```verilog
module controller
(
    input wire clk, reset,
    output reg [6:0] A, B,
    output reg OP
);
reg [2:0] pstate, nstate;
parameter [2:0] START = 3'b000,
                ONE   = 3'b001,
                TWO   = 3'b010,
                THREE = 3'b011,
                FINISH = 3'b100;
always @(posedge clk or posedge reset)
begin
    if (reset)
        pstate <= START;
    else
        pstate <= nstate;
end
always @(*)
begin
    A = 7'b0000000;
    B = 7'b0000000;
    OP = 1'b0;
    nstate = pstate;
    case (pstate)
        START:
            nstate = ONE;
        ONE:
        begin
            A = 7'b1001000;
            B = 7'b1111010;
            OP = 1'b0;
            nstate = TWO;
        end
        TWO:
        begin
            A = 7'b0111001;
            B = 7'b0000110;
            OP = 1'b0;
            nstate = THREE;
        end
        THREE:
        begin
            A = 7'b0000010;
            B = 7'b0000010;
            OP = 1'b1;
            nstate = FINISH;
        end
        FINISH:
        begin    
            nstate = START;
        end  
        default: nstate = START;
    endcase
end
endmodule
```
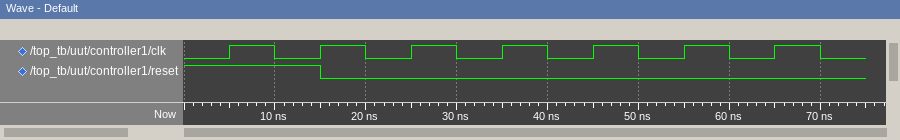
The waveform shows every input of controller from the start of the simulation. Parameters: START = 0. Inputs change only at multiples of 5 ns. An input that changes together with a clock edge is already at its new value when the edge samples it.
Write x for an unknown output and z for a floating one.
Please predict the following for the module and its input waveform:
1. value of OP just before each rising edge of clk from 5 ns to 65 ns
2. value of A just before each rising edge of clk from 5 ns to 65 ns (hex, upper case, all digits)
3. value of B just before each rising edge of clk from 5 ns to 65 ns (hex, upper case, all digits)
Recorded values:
0 0 0 0 1 0 0
00, 00, 48, 39, 02, 00, 00
00, 00, 7A, 06, 02, 00, 00
